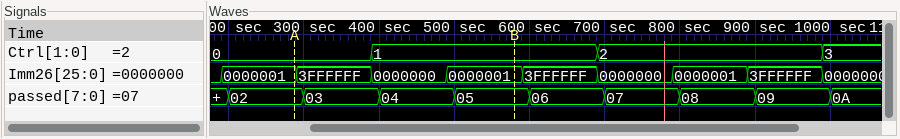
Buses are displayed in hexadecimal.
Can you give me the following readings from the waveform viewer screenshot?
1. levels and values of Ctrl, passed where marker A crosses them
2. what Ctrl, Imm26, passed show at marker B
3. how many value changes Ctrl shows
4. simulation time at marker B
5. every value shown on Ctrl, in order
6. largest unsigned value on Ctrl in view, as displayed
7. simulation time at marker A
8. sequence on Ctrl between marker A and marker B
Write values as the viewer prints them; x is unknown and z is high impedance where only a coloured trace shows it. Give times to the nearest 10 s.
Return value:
Ctrl=0, passed=02
Ctrl=1, Imm26=0000001, passed=05
3
580 s
0, 1, 2, 3
3
290 s
0, 1
